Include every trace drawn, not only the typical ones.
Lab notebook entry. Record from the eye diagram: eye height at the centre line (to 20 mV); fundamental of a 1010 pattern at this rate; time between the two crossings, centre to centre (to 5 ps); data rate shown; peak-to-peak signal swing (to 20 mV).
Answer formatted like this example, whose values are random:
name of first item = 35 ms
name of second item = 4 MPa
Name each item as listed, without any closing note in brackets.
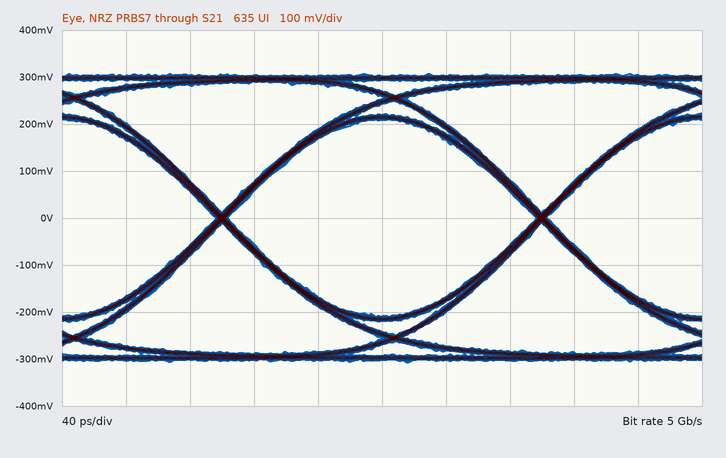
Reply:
eye height at the centre line = 420 mV
fundamental of a 1010 pattern at this rate = 2.5 GHz
time between the two crossings, centre to centre = 200 ps
data rate shown = 5 Gb/s
peak-to-peak signal swing = 620 mV
